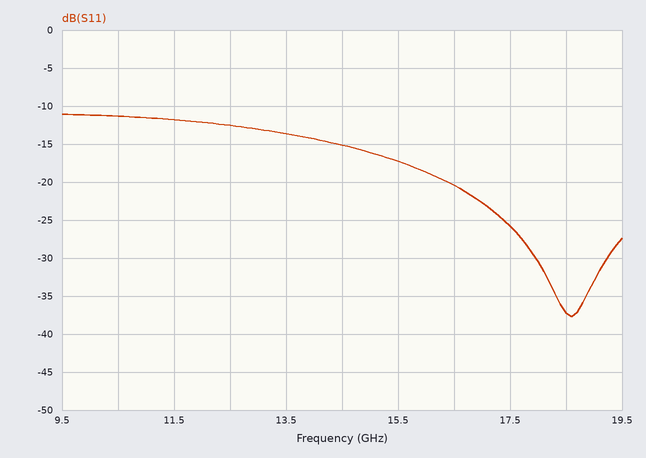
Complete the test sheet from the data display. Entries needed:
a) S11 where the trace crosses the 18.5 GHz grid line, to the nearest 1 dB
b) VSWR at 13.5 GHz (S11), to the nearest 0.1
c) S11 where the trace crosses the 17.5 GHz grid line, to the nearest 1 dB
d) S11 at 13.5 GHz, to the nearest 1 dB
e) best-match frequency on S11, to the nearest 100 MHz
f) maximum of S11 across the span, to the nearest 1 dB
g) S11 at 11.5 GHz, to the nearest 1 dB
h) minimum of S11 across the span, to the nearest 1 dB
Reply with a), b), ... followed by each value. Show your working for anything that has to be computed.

a) -37 dB
b) |Γ| = 10^(-14/20) = 0.1995; VSWR = (1 + 0.1995)/(1 − 0.1995) ≈ 1.5
c) -26 dB
d) -14 dB
e) 18.6 GHz
f) -11 dB
g) -12 dB
h) -38 dB
